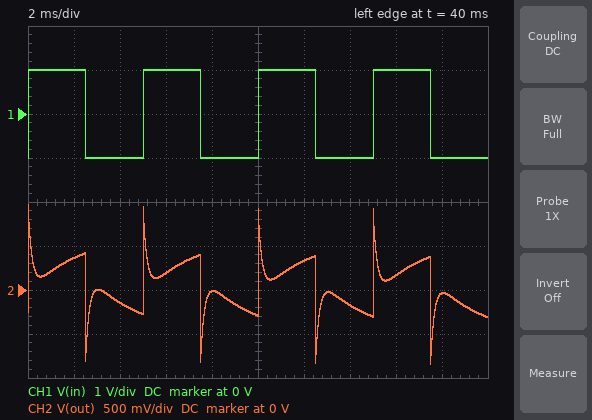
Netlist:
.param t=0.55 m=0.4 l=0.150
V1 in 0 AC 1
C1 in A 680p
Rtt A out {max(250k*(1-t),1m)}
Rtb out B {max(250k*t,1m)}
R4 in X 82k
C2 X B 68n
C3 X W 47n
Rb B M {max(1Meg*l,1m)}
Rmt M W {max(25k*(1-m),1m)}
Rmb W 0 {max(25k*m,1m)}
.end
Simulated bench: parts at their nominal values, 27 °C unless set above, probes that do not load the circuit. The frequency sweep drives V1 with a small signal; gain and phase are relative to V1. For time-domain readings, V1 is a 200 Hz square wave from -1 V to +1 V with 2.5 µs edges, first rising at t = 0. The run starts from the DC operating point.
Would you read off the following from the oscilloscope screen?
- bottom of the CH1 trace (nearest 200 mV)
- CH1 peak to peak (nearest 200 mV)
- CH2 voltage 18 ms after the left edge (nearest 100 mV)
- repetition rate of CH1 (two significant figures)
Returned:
-1.0 V
2.0 V
0 V
200 Hz
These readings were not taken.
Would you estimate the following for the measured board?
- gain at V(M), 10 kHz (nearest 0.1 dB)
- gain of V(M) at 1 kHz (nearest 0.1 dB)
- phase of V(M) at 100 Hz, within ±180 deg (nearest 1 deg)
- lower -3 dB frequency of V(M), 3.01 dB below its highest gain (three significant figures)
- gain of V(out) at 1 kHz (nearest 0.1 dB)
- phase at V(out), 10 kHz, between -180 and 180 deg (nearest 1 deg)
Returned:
-17.1 dB
-18.0 dB
5 deg
14.8 Hz
-7.1 dB
4 deg
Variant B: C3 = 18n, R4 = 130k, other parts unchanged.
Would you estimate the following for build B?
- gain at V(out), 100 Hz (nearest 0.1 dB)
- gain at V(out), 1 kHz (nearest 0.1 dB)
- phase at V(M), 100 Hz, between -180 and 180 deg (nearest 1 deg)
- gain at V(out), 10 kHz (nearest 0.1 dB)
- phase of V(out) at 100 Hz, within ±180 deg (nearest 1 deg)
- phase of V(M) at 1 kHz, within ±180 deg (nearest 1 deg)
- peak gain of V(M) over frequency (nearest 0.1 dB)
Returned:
-7.8 dB
-7.7 dB
1 deg
-4.5 dB
-22 deg
10 deg
-19.6 dB
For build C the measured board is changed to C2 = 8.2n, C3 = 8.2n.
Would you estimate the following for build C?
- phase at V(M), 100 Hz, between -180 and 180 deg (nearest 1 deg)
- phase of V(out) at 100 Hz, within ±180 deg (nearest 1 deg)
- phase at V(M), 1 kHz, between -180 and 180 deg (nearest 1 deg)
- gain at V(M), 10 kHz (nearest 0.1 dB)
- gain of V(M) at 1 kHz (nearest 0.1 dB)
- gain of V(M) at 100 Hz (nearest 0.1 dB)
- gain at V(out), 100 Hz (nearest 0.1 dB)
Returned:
32 deg
24 deg
9 deg
-17.1 dB
-18.1 dB
-19.9 dB
-5.1 dB
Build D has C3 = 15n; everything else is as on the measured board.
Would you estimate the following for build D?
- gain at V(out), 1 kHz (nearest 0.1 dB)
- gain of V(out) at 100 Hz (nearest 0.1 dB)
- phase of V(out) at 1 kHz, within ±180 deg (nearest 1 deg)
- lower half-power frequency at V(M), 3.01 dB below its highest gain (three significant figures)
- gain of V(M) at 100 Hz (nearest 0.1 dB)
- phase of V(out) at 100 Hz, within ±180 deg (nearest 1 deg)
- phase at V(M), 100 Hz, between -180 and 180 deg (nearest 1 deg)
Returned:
-7.6 dB
-4.8 dB
23 deg
27.8 Hz
-19.7 dB
-15 deg
7 deg
